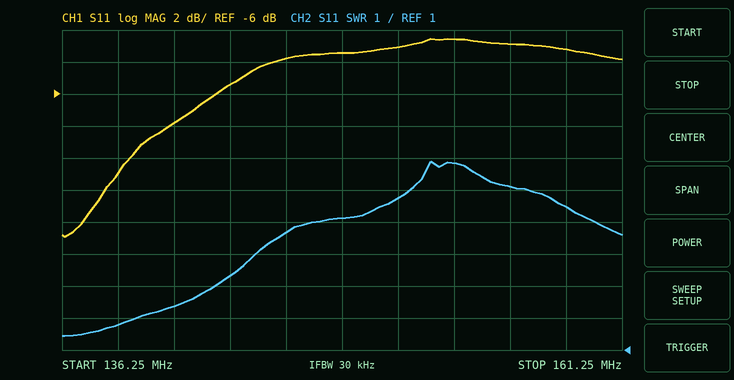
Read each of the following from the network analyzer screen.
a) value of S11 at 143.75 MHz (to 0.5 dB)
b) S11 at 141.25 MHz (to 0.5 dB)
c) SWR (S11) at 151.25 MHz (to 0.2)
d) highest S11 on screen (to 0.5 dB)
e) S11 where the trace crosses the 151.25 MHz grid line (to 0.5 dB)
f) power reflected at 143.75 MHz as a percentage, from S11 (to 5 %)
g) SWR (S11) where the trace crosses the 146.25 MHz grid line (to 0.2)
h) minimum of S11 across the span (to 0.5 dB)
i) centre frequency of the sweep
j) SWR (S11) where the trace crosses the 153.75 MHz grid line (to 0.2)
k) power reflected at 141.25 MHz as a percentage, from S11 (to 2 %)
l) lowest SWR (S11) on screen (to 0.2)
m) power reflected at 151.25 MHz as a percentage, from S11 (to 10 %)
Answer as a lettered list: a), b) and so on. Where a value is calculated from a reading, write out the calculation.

a) -5.5 dB
b) -8.0 dB
c) 5.8
d) -2.5 dB
e) -3.0 dB
f) 10^(-5.5/10) ≈ 28.2 %, so 30 % to the nearest 5 %
g) 4.6
h) -15.0 dB
i) 148.75 MHz
j) 6.8
k) 10^(-8/10) ≈ 16 %
l) 1.4
m) 10^(-3/10) ≈ 50 %
